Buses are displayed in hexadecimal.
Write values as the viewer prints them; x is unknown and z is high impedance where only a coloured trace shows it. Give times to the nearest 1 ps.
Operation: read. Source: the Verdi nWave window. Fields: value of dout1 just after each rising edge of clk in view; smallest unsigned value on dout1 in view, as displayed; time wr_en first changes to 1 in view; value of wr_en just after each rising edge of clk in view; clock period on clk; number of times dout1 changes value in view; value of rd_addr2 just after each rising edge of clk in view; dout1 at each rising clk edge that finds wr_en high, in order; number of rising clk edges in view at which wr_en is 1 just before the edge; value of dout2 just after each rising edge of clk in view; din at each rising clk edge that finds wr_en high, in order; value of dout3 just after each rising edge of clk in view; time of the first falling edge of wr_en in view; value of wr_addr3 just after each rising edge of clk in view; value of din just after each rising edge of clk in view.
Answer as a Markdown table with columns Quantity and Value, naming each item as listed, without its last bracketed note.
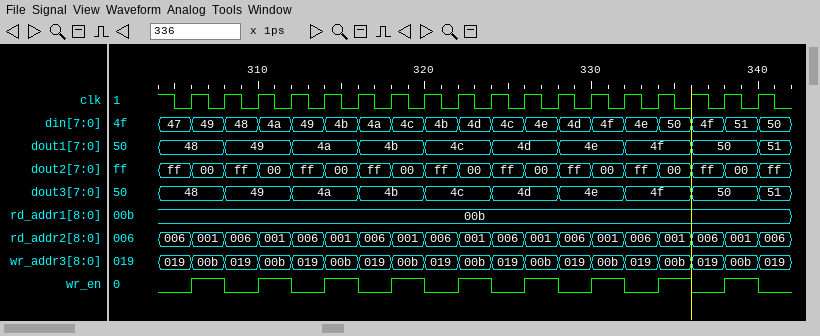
| Quantity | Value |
|---|---|
| value of dout1 just after each rising edge of clk in view | 48, 49, 49, 4a, 4a, 4b, 4b, 4c, 4c, 4d, 4d, 4e, 4e, 4f, 4f, 50, 50, 51 |
| smallest unsigned value on dout1 in view, as displayed | 48 |
| time wr_en first changes to 1 in view | 306 ps |
| value of wr_en just after each rising edge of clk in view | 1 0 1 0 1 0 1 0 1 0 1 0 1 0 1 0 1 0 |
| clock period on clk | 2 ps |
| number of times dout1 changes value in view | 9 |
| value of rd_addr2 just after each rising edge of clk in view | 001, 006, 001, 006, 001, 006, 001, 006, 001, 006, 001, 006, 001, 006, 001, 006, 001, 006 |
| dout1 at each rising clk edge that finds wr_en high, in order | 48, 49, 4a, 4b, 4c, 4d, 4e, 4f, 50 |
| number of rising clk edges in view at which wr_en is 1 just before the edge | 9 |
| value of dout2 just after each rising edge of clk in view | 00, ff, 00, ff, 00, ff, 00, ff, 00, ff, 00, ff, 00, ff, 00, ff, 00, ff |
| din at each rising clk edge that finds wr_en high, in order | 49, 4a, 4b, 4c, 4d, 4e, 4f, 50, 51 |
| value of dout3 just after each rising edge of clk in view | 48, 49, 49, 4a, 4a, 4b, 4b, 4c, 4c, 4d, 4d, 4e, 4e, 4f, 4f, 50, 50, 51 |
| time of the first falling edge of wr_en in view | 308 ps |
| value of wr_addr3 just after each rising edge of clk in view | 00b, 019, 00b, 019, 00b, 019, 00b, 019, 00b, 019, 00b, 019, 00b, 019, 00b, 019, 00b, 019 |
| value of din just after each rising edge of clk in view | 49, 48, 4a, 49, 4b, 4a, 4c, 4b, 4d, 4c, 4e, 4d, 4f, 4e, 50, 4f, 51, 50 |
